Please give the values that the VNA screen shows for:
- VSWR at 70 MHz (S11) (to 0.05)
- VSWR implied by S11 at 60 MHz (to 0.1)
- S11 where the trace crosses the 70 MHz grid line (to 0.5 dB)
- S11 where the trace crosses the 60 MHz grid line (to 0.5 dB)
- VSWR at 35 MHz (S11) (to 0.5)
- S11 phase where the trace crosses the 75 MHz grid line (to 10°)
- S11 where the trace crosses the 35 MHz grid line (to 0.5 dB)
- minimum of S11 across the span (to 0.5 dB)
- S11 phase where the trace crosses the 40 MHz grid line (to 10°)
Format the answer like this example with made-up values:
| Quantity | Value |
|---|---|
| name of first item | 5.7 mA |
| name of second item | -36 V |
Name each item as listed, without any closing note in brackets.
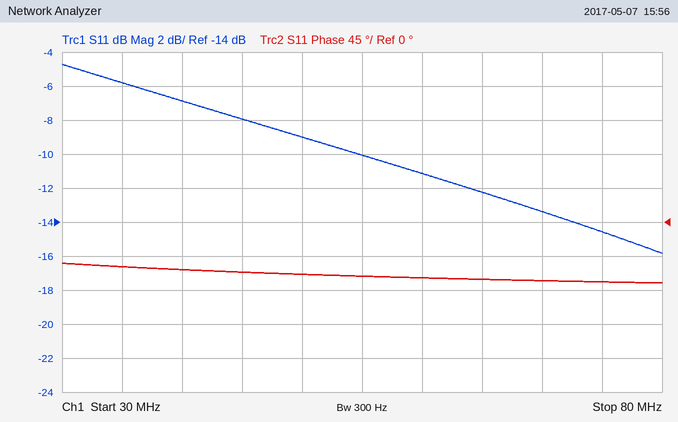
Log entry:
| Quantity | Value |
|---|---|
| VSWR at 70 MHz (S11) | 1.55 |
| VSWR implied by S11 at 60 MHz | 1.8 |
| S11 where the trace crosses the 70 MHz grid line | -13.5 dB |
| S11 where the trace crosses the 60 MHz grid line | -11.0 dB |
| VSWR at 35 MHz (S11) | 3.0 |
| S11 phase where the trace crosses the 75 MHz grid line | -80° |
| S11 where the trace crosses the 35 MHz grid line | -6.0 dB |
| minimum of S11 across the span | -16.0 dB |
| S11 phase where the trace crosses the 40 MHz grid line | -60° |
